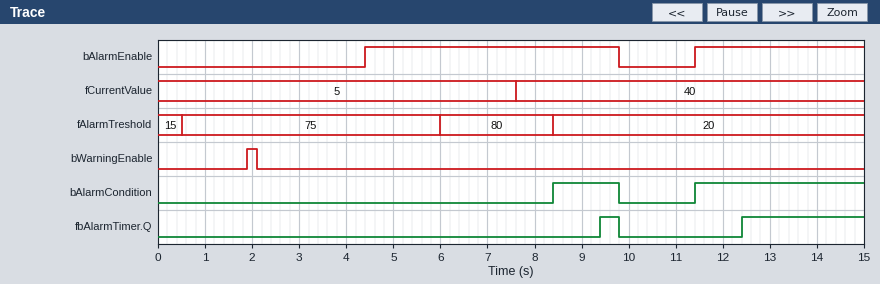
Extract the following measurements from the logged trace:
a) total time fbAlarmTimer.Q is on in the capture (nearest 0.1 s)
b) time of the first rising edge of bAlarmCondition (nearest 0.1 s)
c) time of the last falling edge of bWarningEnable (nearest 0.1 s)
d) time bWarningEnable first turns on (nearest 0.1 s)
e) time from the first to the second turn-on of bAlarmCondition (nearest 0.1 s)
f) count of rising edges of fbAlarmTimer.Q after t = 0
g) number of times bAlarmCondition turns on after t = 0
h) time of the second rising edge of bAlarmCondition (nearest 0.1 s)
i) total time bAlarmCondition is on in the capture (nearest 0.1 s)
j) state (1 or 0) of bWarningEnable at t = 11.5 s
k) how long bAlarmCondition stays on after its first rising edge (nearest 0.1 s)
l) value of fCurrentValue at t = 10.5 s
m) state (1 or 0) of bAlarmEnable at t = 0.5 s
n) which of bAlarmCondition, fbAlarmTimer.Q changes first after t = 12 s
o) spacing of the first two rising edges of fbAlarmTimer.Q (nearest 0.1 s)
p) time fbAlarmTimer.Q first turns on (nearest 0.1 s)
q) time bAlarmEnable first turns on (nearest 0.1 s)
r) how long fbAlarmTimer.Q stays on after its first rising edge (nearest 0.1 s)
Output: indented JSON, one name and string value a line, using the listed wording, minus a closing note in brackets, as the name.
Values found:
{
  "total time fbAlarmTimer.Q is on in the capture": "3.0 s",
  "time of the first rising edge of bAlarmCondition": "8.4 s",
  "time of the last falling edge of bWarningEnable": "2.1 s",
  "time bWarningEnable first turns on": "1.9 s",
  "time from the first to the second turn-on of bAlarmCondition": "3.0 s",
  "count of rising edges of fbAlarmTimer.Q after t = 0": "2",
  "number of times bAlarmCondition turns on after t = 0": "2",
  "time of the second rising edge of bAlarmCondition": "11.4 s",
  "total time bAlarmCondition is on in the capture": "5.0 s",
  "state (1 or 0) of bWarningEnable at t = 11.5 s": "0",
  "how long bAlarmCondition stays on after its first rising edge": "1.4 s",
  "value of fCurrentValue at t = 10.5 s": "40",
  "state (1 or 0) of bAlarmEnable at t = 0.5 s": "0",
  "which of bAlarmCondition, fbAlarmTimer.Q changes first after t = 12 s": "fbAlarmTimer.Q",
  "spacing of the first two rising edges of fbAlarmTimer.Q": "3.0 s",
  "time fbAlarmTimer.Q first turns on": "9.4 s",
  "time bAlarmEnable first turns on": "4.4 s",
  "how long fbAlarmTimer.Q stays on after its first rising edge": "0.4 s"
}
